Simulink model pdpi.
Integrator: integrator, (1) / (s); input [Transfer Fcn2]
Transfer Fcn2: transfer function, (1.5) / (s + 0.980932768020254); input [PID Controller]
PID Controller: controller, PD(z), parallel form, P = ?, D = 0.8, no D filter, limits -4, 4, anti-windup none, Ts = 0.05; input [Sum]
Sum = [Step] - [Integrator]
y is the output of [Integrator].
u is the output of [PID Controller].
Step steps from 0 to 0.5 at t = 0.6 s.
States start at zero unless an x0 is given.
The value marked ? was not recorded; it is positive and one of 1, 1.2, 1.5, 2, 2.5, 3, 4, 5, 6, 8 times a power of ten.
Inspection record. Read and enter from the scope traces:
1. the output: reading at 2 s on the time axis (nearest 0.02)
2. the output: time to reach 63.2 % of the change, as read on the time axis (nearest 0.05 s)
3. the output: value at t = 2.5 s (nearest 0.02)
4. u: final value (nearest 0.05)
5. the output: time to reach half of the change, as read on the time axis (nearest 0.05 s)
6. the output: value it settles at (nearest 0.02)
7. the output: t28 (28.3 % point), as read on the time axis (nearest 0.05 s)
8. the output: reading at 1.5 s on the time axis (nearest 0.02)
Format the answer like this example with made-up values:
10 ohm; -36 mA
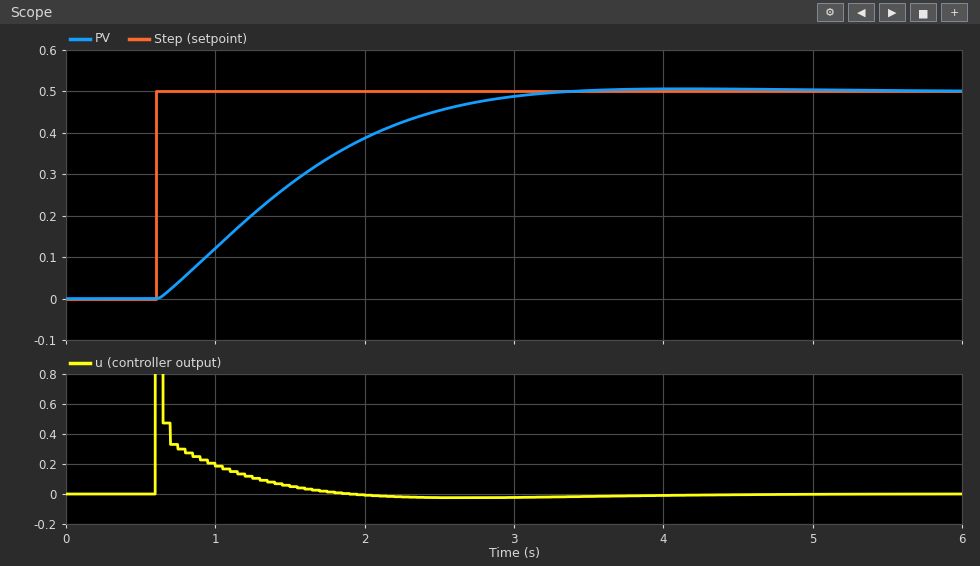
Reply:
0.38; 1.65 s; 0.46; 0.00; 1.40 s; 0.50; 1.05 s; 0.28
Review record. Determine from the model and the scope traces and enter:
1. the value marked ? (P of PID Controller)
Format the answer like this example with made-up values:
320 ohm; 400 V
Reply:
1.2
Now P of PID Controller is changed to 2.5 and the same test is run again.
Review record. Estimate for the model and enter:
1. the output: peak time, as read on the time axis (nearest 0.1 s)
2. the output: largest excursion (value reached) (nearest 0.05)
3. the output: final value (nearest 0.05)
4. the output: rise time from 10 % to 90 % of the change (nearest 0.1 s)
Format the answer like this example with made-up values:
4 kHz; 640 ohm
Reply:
2.4 s; 0.55; 0.50; 0.8 s
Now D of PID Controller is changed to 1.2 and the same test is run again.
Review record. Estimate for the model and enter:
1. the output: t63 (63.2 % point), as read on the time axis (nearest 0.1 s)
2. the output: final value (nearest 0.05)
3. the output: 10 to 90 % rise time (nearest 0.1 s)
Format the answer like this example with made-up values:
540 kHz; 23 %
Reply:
1.9 s; 0.50; 2.5 s
